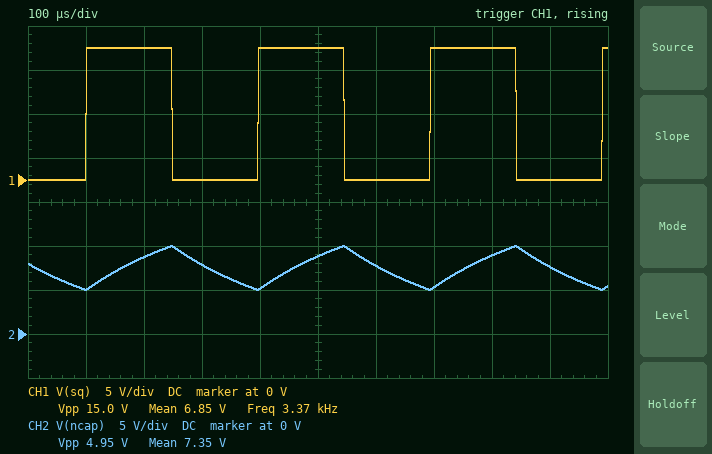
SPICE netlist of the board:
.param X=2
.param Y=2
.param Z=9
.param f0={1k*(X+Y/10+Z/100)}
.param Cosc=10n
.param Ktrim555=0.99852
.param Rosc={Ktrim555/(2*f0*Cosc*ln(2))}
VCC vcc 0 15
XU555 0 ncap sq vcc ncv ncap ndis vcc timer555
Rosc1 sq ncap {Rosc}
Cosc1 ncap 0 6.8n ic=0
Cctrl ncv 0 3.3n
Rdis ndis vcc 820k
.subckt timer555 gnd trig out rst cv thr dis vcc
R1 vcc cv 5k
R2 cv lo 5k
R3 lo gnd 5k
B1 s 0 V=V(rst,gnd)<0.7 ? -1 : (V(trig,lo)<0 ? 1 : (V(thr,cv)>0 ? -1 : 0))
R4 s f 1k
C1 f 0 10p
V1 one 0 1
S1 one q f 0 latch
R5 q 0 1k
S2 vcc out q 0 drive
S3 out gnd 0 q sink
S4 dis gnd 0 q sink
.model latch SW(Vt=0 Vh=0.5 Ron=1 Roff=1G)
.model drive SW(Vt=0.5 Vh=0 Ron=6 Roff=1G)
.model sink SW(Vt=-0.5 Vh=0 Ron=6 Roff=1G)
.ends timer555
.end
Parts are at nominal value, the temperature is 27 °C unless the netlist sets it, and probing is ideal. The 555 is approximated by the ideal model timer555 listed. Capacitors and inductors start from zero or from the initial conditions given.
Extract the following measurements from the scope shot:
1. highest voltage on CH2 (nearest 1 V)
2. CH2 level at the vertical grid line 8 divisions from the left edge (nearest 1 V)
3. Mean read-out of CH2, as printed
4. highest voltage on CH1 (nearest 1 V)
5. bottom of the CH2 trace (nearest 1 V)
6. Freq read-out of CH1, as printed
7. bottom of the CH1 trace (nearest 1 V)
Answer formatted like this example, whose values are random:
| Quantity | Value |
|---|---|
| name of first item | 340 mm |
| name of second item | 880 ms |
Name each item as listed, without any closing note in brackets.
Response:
| Quantity | Value |
|---|---|
| highest voltage on CH2 | 10 V |
| CH2 level at the vertical grid line 8 divisions from the left edge | 9 V |
| Mean read-out of CH2, as printed | 7.35 V |
| highest voltage on CH1 | 15 V |
| bottom of the CH2 trace | 5 V |
| Freq read-out of CH1, as printed | 3.37 kHz |
| bottom of the CH1 trace | 0 V |
